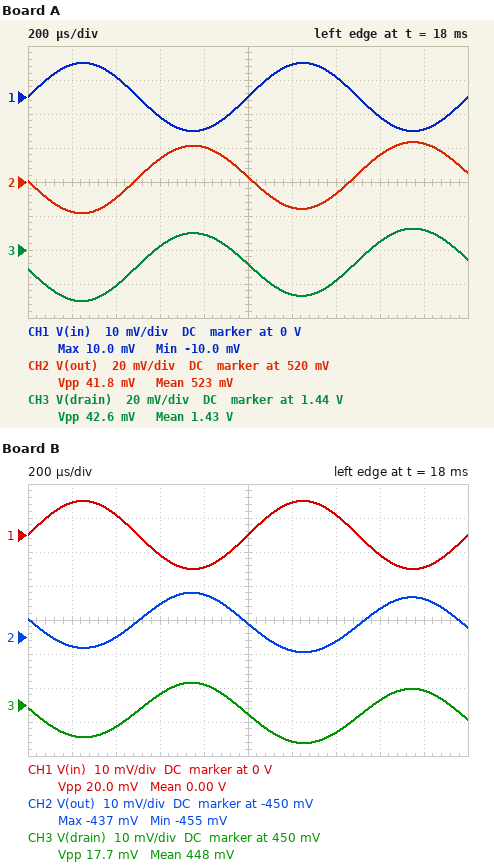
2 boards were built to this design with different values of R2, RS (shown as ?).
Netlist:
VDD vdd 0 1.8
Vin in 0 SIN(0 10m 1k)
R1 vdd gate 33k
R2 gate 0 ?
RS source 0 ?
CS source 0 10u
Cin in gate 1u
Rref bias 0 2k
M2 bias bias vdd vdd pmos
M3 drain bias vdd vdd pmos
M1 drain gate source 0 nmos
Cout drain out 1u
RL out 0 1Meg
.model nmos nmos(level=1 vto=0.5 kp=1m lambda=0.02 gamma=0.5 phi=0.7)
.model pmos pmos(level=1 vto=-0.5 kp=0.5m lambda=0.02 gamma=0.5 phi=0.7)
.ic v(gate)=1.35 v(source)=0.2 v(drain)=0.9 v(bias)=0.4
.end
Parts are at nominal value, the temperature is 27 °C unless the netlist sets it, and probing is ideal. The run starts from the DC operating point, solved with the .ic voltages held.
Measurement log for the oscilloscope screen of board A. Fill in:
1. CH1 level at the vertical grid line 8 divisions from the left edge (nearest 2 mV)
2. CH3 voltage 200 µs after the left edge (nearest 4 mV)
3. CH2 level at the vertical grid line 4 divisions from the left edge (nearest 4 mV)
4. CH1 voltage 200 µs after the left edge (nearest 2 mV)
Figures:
-6 mV
1.412 V
540 mV
10 mV
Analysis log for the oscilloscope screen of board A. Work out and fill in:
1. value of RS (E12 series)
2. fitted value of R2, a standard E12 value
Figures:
2.7 kΩ
120 kΩ
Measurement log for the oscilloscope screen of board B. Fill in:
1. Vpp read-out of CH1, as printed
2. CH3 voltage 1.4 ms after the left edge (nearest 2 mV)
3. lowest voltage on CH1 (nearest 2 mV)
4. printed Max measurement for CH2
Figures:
20.0 mV
442 mV
-10 mV
-437 mV
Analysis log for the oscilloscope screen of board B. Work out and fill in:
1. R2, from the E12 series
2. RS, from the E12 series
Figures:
120 kΩ
470 Ω
